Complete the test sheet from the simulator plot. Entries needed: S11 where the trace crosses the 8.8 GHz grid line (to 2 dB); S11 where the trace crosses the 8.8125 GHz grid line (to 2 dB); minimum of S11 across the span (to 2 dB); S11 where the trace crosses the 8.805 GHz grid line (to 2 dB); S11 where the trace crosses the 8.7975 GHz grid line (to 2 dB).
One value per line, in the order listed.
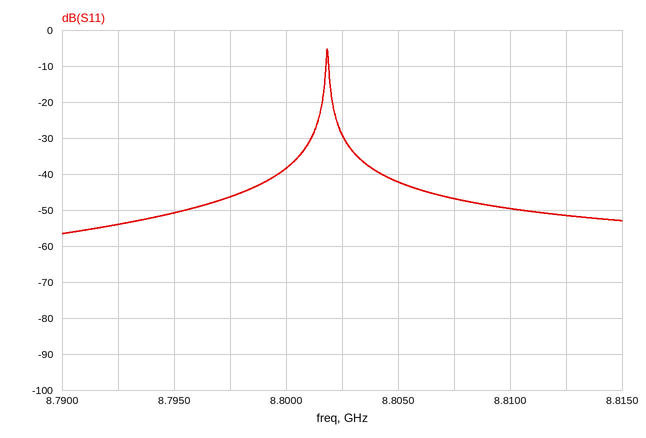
-38 dB
-52 dB
-56 dB
-42 dB
-46 dB
